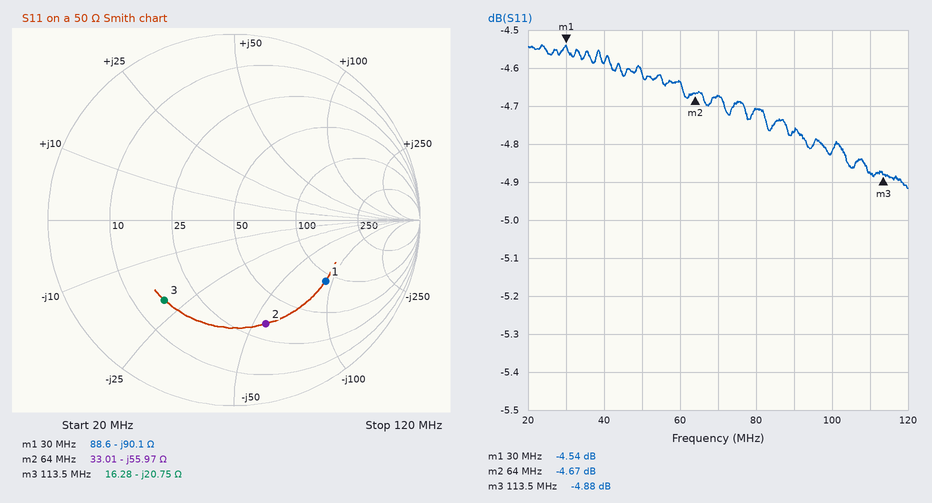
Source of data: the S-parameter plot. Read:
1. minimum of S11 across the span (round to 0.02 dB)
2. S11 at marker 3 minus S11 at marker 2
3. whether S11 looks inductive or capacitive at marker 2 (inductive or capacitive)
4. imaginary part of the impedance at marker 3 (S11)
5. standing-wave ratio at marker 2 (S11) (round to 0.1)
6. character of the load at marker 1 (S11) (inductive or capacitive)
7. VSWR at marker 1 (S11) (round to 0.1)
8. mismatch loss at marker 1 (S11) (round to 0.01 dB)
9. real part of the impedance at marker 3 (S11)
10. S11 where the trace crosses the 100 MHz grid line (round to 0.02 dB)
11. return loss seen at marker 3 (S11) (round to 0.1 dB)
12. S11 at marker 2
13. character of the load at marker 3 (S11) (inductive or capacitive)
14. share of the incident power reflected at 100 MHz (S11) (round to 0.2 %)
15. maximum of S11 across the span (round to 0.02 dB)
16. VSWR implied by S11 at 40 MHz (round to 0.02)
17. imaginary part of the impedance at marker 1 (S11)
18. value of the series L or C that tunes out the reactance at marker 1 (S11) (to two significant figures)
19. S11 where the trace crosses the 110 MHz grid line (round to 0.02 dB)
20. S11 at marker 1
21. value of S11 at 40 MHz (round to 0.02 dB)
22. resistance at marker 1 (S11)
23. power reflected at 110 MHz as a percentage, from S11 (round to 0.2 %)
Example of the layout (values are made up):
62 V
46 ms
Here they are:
-4.92 dB
-0.21 dB
capacitive
-20.75 Ω
3.8
capacitive
3.9
1.88 dB
16.28 Ω
-4.82 dB
4.9 dB
-4.67 dB
capacitive
33.0 %
-4.54 dB
3.88
-90.1 Ω
480 nH
-4.88 dB
-4.54 dB
-4.58 dB
88.6 Ω
32.6 %
